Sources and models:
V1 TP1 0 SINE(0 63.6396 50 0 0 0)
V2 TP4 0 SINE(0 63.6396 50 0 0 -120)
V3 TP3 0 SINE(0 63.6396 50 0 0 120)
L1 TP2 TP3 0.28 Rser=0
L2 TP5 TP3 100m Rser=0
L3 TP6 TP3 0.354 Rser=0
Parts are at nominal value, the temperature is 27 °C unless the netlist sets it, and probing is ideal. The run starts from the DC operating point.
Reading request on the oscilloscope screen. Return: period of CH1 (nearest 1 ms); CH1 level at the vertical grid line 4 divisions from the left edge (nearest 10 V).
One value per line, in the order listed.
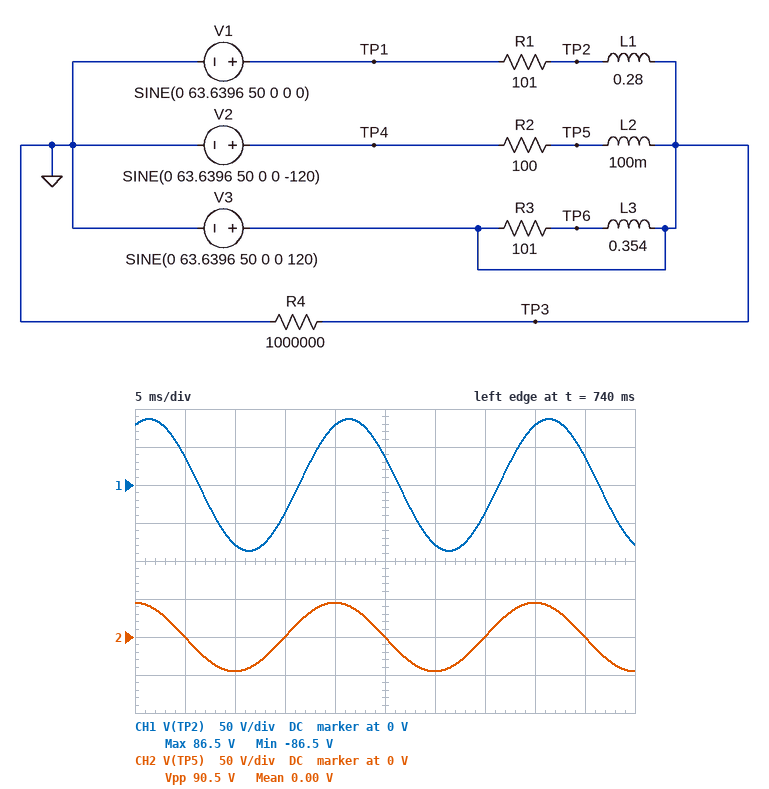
20 ms
80 V
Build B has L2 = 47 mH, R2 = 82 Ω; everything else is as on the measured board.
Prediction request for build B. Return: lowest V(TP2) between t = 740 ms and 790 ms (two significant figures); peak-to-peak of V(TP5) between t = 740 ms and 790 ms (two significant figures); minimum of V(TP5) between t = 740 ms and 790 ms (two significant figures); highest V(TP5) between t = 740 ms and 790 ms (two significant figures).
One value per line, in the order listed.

-87 V
110 V
-53 V
53 V
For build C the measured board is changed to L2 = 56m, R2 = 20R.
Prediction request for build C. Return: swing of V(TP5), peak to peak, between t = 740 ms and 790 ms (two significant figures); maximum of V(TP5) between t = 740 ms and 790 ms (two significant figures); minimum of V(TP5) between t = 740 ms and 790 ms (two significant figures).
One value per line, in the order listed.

48 V
24 V
-24 V
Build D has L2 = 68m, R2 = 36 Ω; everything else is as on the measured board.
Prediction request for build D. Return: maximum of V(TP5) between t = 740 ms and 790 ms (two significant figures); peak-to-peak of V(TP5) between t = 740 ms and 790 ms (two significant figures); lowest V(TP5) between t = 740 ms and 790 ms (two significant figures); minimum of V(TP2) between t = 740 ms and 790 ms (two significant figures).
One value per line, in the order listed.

31 V
62 V
-31 V
-87 V
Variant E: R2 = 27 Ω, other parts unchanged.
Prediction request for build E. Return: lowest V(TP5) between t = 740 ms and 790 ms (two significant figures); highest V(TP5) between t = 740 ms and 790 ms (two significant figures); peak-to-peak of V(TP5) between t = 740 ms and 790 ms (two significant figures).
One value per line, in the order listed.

-24 V
24 V
48 V
